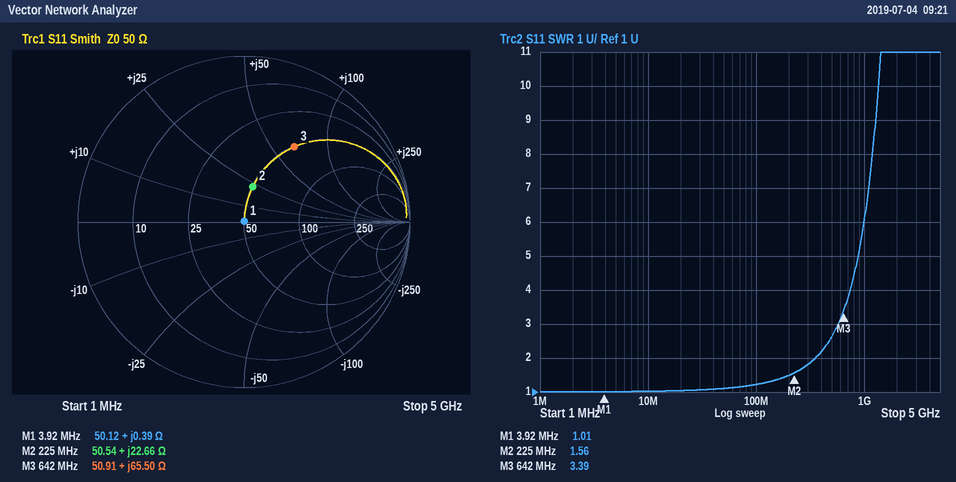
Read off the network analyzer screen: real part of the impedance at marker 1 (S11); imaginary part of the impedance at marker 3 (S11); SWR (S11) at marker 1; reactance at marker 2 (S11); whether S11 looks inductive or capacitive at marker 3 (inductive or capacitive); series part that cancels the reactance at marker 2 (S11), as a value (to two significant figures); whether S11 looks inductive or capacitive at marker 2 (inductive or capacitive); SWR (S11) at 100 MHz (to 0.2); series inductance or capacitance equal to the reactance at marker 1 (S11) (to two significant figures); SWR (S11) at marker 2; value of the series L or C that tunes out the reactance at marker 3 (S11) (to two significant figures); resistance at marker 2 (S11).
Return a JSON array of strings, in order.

["50.12 Ω", "+65.50 Ω", "1.01", "+22.66 Ω", "inductive", "31 pF", "inductive", "1.2", "16 nH", "1.56", "3.8 pF", "50.54 Ω"]
